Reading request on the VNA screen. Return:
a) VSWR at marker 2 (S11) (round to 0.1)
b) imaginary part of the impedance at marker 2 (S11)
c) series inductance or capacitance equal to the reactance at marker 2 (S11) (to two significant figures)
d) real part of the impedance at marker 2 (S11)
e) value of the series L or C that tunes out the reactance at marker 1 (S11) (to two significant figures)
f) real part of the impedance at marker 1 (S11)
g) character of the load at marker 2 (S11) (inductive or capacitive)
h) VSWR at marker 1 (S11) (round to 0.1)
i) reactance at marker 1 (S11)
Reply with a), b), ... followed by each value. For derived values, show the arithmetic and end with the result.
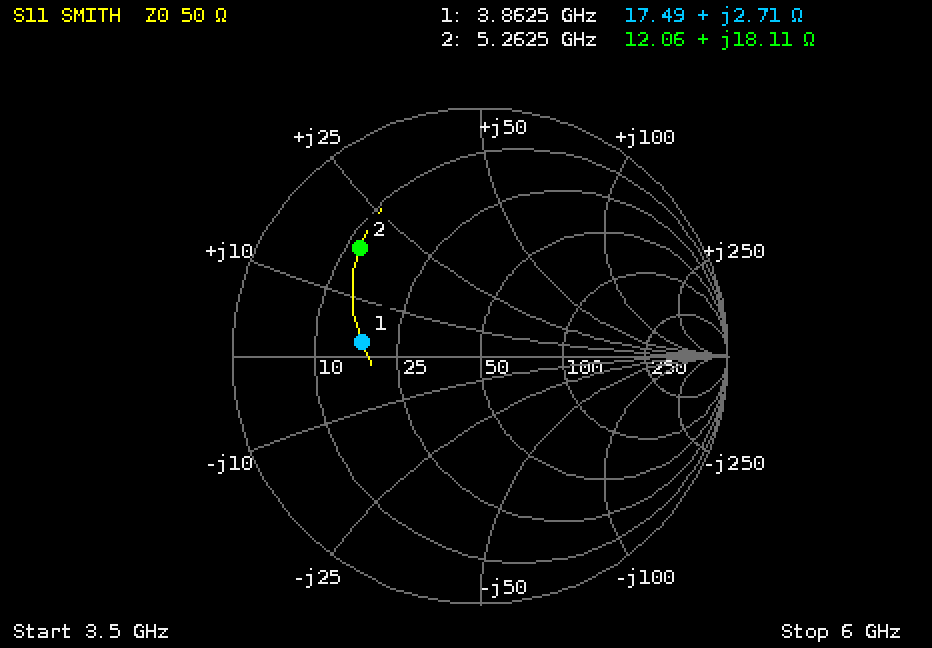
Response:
a) 4.7
b) +18.11 Ω
c) L = 18.11 Ω/(2π × 5.2625 GHz) ≈ 548 pH, so 550 pH to two significant figures
d) 12.06 Ω
e) C = 1/(2π × 3.8625 GHz × 2.71 Ω) ≈ 15 pF
f) 17.49 Ω
g) inductive
h) 2.9
i) +2.71 Ω
